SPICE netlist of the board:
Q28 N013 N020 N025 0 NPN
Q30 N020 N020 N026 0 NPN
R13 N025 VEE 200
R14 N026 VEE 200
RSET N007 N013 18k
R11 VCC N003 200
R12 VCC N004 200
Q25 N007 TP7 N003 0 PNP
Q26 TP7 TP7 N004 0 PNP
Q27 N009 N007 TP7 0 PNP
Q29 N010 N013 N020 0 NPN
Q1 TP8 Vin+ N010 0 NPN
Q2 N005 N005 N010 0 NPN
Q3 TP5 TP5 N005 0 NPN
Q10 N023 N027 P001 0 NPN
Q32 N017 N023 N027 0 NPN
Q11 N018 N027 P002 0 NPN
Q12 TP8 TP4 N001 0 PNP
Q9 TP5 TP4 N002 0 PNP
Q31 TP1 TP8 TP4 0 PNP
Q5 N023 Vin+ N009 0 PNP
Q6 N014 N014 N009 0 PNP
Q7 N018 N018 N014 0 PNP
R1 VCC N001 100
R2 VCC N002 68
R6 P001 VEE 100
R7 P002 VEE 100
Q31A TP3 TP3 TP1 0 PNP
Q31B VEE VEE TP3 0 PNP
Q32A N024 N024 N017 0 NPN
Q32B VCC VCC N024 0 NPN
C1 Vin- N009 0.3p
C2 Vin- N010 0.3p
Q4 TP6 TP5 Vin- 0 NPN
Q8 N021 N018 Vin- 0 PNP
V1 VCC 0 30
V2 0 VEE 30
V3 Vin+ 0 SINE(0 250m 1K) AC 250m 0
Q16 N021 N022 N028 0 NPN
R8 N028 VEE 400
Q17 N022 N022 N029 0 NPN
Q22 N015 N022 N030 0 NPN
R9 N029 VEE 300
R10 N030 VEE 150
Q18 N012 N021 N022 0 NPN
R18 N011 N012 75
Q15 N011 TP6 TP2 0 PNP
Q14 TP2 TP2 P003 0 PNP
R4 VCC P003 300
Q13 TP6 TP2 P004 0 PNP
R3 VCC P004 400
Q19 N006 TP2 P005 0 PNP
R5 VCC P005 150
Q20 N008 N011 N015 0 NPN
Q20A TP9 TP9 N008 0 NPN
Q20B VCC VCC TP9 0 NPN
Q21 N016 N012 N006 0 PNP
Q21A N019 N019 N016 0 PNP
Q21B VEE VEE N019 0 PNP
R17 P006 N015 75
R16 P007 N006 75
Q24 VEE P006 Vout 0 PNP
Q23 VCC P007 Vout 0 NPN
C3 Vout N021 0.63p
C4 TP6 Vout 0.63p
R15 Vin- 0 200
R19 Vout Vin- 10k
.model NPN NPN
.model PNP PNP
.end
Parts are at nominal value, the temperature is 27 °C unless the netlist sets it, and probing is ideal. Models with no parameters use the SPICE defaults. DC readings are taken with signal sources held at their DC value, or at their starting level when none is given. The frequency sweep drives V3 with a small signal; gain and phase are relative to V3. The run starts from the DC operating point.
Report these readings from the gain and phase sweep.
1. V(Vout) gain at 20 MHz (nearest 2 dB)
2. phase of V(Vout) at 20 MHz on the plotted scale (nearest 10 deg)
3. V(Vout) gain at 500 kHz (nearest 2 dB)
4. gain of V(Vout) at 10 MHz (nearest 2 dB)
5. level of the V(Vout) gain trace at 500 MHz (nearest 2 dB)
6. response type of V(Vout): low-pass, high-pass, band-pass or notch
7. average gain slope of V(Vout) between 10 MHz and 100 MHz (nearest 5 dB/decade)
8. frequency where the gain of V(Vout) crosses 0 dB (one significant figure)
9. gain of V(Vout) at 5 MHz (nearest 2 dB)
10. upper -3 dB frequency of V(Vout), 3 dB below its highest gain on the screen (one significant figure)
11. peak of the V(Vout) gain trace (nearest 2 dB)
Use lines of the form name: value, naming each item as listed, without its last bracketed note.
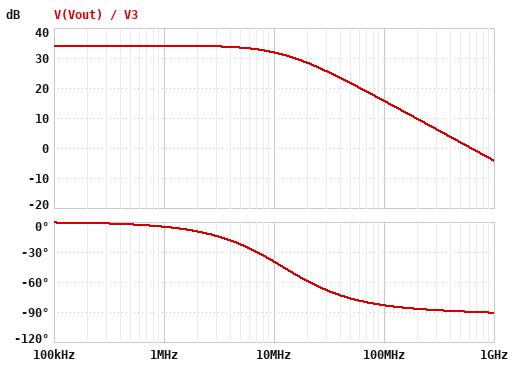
V(Vout) gain at 20 MHz: 28 dB
phase of V(Vout) at 20 MHz on the plotted scale: -60 deg
V(Vout) gain at 500 kHz: 34 dB
gain of V(Vout) at 10 MHz: 32 dB
level of the V(Vout) gain trace at 500 MHz: 2 dB
response type of V(Vout): low-pass, high-pass, band-pass or notch: low-pass
average gain slope of V(Vout) between 10 MHz and 100 MHz: -15 dB/decade
frequency where the gain of V(Vout) crosses 0 dB: 600 MHz
gain of V(Vout) at 5 MHz: 34 dB
upper -3 dB frequency of V(Vout), 3 dB below its highest gain on the screen: 10 MHz
peak of the V(Vout) gain trace: 34 dB
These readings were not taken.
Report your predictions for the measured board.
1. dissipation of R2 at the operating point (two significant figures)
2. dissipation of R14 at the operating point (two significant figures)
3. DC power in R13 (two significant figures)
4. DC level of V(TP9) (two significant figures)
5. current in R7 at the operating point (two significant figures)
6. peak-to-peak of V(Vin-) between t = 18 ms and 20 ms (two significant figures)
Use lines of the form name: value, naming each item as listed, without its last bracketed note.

dissipation of R2 at the operating point: 220 µW
dissipation of R14 at the operating point: 1.9 mW
DC power in R13: 1.9 mW
DC level of V(TP9): 29 V
current in R7 at the operating point: 1.6 mA
peak-to-peak of V(Vin-) between t = 18 ms and 20 ms: 500 mV
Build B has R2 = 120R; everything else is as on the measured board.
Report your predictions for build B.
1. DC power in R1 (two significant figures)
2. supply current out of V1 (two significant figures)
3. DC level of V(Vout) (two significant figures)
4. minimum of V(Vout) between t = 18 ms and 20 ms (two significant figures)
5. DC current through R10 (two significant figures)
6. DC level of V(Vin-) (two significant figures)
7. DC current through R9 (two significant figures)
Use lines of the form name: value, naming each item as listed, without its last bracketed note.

DC power in R1: 280 µW
supply current out of V1: 19 mA
DC level of V(Vout): -160 mV
minimum of V(Vout) between t = 18 ms and 20 ms: -13 V
DC current through R10: 3.3 mA
DC level of V(Vin-): -3.1 mV
DC current through R9: 1.7 mA
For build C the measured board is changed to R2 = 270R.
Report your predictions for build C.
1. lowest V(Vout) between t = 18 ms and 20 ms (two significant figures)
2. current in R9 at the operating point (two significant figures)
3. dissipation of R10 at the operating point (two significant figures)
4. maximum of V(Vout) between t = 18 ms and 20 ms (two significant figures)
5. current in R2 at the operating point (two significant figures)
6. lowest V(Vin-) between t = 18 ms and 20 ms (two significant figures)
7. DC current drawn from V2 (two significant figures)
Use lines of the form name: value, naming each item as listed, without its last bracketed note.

lowest V(Vout) between t = 18 ms and 20 ms: -14 V
current in R9 at the operating point: 940 µA
dissipation of R10 at the operating point: 470 µW
maximum of V(Vout) between t = 18 ms and 20 ms: 12 V
current in R2 at the operating point: 900 µA
lowest V(Vin-) between t = 18 ms and 20 ms: -270 mV
DC current drawn from V2: 15 mA
